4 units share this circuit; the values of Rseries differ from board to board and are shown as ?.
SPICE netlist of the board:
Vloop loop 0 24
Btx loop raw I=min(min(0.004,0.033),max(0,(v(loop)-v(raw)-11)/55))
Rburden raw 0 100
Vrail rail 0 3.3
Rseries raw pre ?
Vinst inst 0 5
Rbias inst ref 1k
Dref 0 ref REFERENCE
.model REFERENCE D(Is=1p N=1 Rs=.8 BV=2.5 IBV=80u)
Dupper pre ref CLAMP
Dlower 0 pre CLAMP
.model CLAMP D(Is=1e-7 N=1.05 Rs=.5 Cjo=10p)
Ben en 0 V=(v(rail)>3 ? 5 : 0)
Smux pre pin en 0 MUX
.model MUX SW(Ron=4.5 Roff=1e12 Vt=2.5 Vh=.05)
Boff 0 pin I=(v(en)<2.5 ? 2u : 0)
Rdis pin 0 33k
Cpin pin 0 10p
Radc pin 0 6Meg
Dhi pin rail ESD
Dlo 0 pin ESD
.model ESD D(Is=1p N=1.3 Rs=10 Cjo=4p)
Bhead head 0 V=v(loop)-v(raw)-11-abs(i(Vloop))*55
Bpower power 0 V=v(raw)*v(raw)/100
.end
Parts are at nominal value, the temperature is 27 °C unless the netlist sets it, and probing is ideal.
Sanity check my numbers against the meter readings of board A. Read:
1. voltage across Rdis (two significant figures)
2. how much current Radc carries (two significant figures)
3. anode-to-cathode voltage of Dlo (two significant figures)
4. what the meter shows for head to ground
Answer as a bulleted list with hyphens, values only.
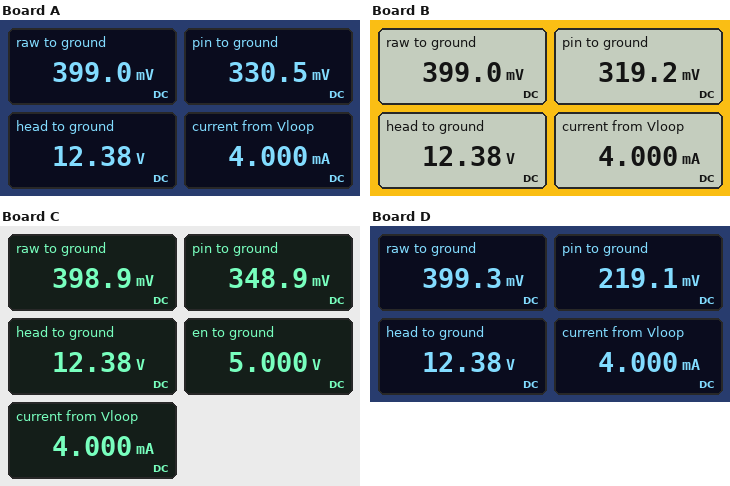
- 330 mV
- 55 nA
- -330 mV
- 12.38 V
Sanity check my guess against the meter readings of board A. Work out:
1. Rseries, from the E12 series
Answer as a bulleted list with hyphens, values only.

- 6.8 kΩ
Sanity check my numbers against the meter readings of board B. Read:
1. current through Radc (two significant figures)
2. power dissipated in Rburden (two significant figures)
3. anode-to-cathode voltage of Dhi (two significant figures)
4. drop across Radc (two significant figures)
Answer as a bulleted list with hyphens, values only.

- 53 nA
- 1.6 mW
- -3.0 V
- 320 mV
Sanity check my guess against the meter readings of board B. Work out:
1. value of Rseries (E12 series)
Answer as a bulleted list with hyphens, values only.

- 8.2 kΩ
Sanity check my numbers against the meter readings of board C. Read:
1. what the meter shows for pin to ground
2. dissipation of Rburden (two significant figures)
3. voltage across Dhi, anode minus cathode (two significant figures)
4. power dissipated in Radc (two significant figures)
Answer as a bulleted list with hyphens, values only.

- 348.9 mV
- 1.6 mW
- -3.0 V
- 20 nW
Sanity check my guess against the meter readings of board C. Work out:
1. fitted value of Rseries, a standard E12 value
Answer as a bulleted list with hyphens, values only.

- 4.7 kΩ
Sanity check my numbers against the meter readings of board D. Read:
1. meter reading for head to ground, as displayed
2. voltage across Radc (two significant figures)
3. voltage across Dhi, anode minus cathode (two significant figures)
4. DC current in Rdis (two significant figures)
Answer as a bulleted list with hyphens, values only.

- 12.38 V
- 220 mV
- -3.1 V
- 6.6 µA
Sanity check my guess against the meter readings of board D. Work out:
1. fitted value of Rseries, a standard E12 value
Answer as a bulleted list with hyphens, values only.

- 27 kΩ
